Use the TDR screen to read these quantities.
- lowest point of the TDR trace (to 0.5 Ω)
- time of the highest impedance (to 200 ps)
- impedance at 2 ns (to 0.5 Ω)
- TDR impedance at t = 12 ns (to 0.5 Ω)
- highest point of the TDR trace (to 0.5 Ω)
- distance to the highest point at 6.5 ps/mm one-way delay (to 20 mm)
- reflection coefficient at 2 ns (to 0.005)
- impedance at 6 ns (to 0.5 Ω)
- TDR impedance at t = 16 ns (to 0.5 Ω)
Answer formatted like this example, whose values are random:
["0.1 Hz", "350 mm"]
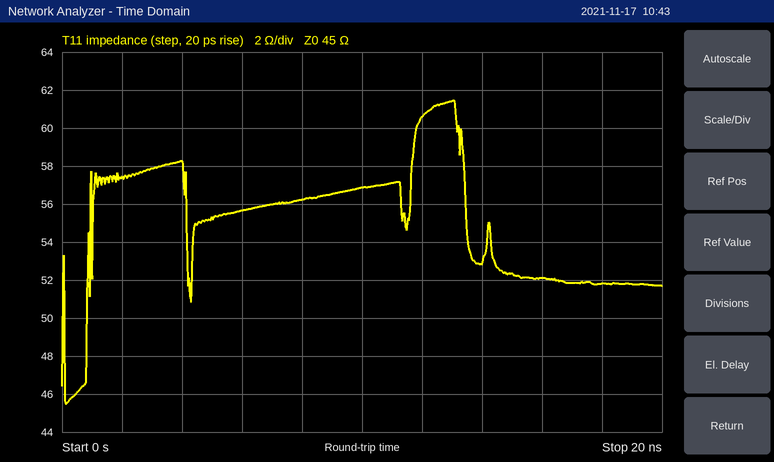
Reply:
["45.5 Ω", "13.0 ns", "57.5 Ω", "60.5 Ω", "61.5 Ω", "1.00 m", "+0.120", "55.5 Ω", "52.0 Ω"]
